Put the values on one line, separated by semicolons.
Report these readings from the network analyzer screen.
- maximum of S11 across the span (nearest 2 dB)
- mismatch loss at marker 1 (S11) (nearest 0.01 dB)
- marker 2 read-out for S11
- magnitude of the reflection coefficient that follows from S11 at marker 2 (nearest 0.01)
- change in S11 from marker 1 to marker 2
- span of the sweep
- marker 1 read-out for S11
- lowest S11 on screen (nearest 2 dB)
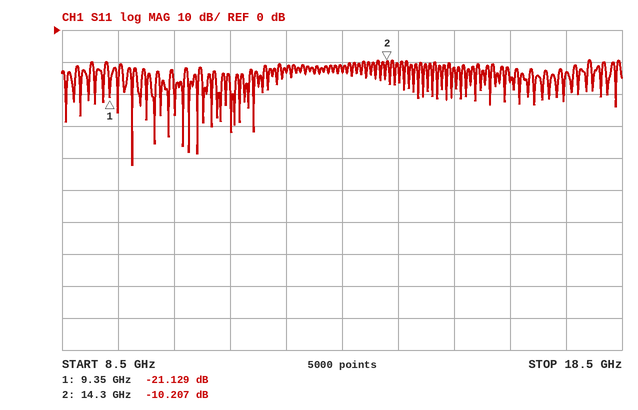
-10 dB; 0.03 dB; -10.207 dB; 0.31; 10.922 dB; 10 GHz; -21.129 dB; -42 dB
